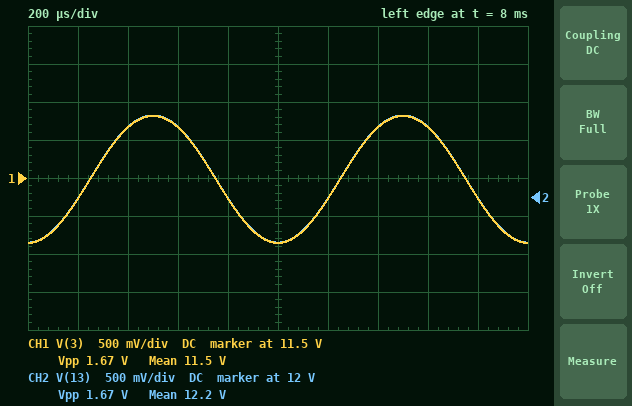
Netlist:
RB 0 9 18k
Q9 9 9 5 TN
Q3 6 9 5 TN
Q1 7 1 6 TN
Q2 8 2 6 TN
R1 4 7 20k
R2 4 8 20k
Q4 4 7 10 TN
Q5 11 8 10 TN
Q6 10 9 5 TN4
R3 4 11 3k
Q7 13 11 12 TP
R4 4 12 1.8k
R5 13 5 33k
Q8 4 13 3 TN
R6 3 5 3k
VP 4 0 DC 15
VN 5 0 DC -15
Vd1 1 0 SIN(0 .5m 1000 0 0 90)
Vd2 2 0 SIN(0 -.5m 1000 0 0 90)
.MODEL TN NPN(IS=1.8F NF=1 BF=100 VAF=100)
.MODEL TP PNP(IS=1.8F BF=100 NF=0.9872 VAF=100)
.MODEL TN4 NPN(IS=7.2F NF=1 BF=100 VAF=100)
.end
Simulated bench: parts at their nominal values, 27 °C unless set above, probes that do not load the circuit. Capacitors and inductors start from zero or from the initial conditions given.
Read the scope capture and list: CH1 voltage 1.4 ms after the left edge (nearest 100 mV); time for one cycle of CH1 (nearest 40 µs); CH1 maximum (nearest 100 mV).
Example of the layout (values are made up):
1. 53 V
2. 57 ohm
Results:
1. 12.2 V
2. 1.00 ms
3. 12.3 V
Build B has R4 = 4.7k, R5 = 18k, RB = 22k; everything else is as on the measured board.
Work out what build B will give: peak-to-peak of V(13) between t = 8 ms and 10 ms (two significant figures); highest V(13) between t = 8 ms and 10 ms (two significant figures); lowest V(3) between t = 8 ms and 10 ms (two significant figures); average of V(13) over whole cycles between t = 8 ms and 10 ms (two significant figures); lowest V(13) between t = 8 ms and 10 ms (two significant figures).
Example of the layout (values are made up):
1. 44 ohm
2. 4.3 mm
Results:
1. 13 V
2. 4.7 V
3. -9.2 V
4. -1.9 V
5. -8.5 V
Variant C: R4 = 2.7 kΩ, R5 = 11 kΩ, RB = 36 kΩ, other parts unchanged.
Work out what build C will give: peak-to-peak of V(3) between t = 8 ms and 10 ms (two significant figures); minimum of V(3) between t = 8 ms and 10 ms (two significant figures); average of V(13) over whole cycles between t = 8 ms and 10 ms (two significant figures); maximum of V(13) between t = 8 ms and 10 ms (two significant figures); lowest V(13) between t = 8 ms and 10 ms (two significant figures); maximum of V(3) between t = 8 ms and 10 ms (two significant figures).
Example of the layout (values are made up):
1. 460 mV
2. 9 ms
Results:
1. 8.2 V
2. -12 V
3. -7.0 V
4. -2.9 V
5. -11 V
6. -3.6 V
